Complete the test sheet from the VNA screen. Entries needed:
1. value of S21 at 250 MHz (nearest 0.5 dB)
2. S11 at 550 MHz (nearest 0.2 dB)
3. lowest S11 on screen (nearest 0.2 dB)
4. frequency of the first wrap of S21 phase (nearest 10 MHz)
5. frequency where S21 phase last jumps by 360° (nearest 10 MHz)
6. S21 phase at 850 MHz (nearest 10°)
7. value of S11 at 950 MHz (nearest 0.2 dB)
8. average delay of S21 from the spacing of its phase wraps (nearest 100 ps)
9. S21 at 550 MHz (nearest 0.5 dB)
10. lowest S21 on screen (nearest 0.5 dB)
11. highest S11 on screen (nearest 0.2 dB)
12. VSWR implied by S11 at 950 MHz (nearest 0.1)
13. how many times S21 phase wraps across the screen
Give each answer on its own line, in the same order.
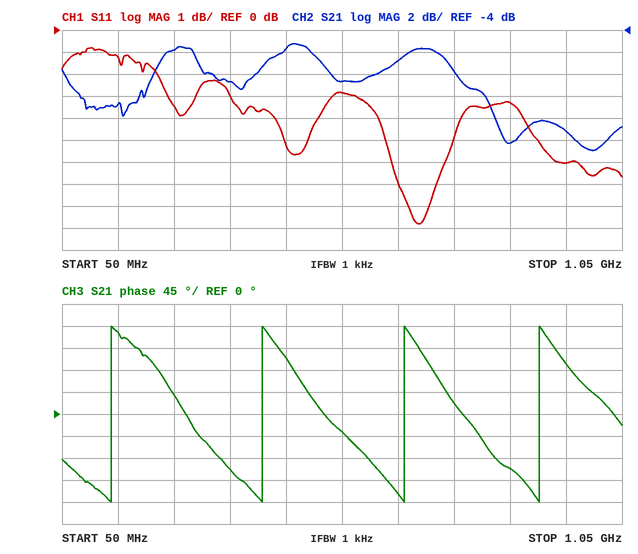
-6.0 dB
-2.8 dB
-8.8 dB
140 MHz
900 MHz
-110°
-6.0 dB
3.9 ns
-8.5 dB
-15.0 dB
-0.8 dB
3.0
4
